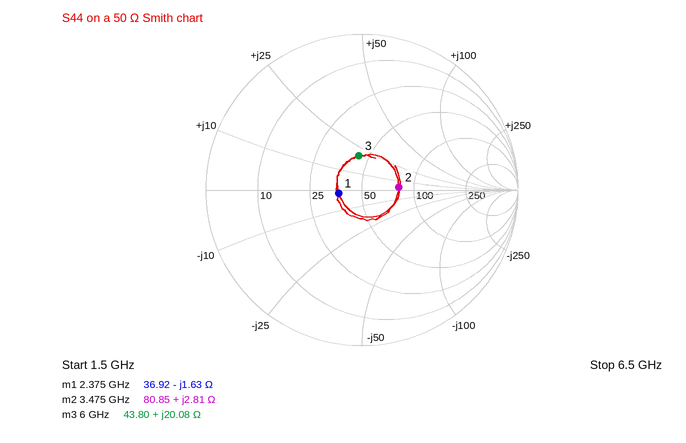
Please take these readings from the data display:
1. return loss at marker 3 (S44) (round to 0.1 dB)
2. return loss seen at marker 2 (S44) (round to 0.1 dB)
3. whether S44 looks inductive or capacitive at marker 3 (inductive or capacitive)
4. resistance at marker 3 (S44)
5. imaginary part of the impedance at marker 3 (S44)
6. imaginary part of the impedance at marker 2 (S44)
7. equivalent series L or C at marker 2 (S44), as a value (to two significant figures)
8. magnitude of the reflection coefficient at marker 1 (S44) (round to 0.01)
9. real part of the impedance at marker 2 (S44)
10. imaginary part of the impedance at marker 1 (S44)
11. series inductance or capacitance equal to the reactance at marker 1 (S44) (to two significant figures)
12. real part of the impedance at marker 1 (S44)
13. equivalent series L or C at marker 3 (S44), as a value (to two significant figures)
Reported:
13.2 dB
12.5 dB
inductive
43.80 Ω
+20.08 Ω
+2.81 Ω
130 pH
0.15
80.85 Ω
-1.63 Ω
41 pF
36.92 Ω
530 pH
